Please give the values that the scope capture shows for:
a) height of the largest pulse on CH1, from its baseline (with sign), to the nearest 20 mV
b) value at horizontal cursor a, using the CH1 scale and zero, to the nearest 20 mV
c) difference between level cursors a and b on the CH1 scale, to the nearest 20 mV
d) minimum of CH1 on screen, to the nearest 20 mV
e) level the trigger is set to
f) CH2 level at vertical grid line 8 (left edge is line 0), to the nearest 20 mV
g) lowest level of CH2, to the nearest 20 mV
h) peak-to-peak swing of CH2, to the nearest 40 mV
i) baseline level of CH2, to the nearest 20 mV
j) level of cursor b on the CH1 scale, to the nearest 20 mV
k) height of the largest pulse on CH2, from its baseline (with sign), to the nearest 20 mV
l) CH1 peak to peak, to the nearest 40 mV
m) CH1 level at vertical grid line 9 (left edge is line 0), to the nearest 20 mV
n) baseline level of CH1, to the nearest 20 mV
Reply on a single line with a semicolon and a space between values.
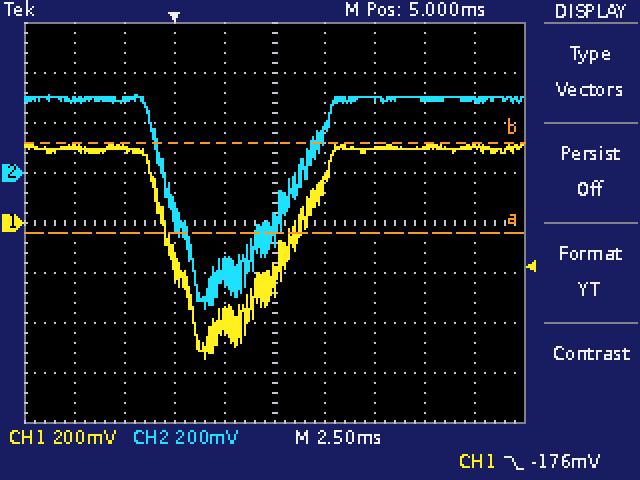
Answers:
-840 mV; -40 mV; 360 mV; -540 mV; -176 mV; 300 mV; -540 mV; 840 mV; 300 mV; 320 mV; -840 mV; 840 mV; 300 mV; 300 mV
